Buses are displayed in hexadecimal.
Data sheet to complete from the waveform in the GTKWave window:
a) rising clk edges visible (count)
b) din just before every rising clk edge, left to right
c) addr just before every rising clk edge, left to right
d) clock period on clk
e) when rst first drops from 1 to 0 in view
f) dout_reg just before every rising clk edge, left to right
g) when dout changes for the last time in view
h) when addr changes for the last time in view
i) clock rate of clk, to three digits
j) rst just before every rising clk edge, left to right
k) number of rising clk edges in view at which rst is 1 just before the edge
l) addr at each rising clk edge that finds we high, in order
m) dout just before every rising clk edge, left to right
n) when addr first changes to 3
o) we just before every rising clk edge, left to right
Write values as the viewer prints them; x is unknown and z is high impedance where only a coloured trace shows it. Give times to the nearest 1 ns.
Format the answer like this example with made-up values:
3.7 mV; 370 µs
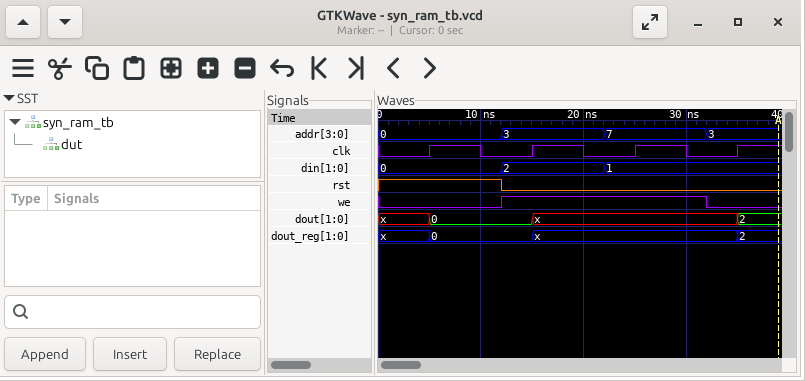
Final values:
4; 0, 2, 1, 1; 0, 3, 7, 3; 10 ns; 12 ns; x, 0, x, x; 35 ns; 32 ns; 100 MHz; 1 0 0 0; 1; 3, 7; x, 0, x, x; 12 ns; 0 1 1 0
